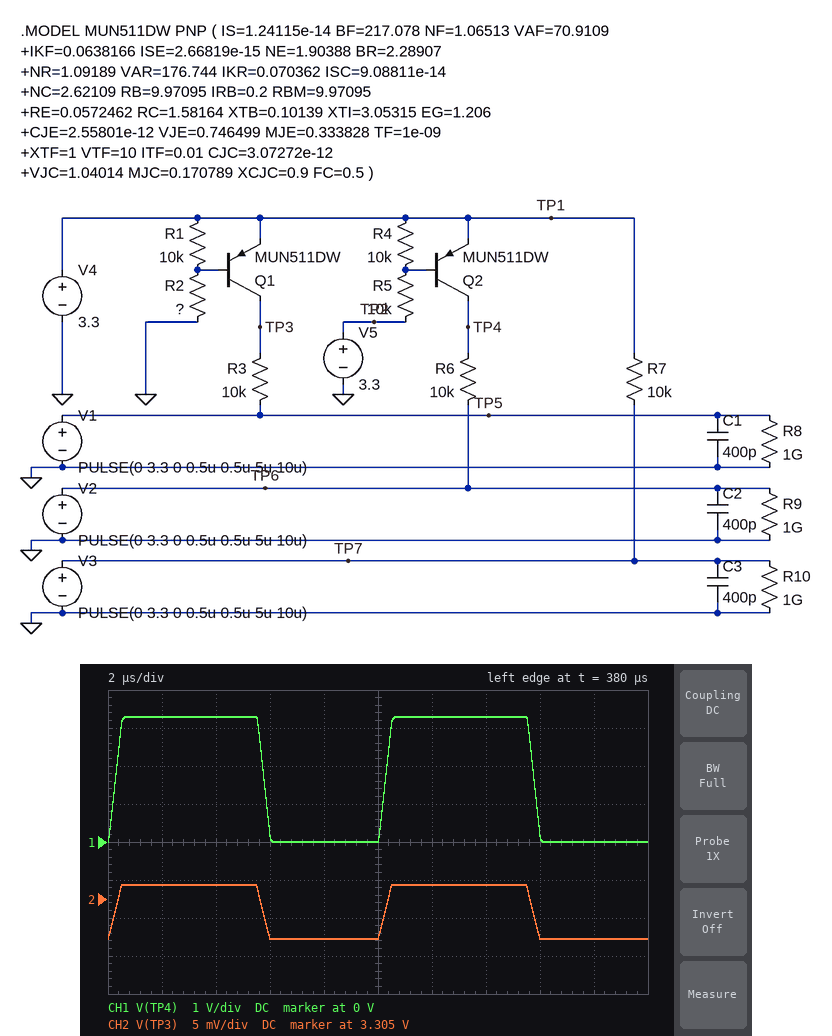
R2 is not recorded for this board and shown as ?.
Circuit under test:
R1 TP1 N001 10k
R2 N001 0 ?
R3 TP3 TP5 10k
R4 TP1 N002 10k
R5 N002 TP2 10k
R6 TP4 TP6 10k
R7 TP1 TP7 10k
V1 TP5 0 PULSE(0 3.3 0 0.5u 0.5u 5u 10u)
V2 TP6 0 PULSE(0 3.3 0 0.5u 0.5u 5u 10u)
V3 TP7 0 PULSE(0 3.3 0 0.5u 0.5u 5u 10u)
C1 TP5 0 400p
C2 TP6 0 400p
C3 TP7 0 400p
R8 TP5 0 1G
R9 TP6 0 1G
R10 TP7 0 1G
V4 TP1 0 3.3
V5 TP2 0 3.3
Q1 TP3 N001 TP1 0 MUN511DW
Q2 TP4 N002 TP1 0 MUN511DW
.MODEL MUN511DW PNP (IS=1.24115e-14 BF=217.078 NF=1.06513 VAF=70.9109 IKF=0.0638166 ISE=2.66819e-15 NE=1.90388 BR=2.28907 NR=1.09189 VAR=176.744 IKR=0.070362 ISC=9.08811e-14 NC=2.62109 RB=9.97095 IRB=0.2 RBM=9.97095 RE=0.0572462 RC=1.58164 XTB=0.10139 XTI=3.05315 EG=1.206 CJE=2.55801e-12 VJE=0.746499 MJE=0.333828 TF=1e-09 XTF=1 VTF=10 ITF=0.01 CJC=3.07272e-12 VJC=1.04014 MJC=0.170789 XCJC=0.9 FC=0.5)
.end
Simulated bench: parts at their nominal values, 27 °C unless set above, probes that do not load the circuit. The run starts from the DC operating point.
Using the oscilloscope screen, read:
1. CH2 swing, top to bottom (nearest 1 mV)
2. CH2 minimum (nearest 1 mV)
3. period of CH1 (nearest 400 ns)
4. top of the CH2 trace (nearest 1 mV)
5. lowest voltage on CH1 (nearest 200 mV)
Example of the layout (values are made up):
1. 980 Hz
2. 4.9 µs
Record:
1. 7 mV
2. 3.300 V
3. 10.0 µs
4. 3.307 V
5. 0 V
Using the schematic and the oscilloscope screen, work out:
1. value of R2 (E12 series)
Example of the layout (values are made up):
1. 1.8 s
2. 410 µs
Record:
1. 5.6 kΩ
